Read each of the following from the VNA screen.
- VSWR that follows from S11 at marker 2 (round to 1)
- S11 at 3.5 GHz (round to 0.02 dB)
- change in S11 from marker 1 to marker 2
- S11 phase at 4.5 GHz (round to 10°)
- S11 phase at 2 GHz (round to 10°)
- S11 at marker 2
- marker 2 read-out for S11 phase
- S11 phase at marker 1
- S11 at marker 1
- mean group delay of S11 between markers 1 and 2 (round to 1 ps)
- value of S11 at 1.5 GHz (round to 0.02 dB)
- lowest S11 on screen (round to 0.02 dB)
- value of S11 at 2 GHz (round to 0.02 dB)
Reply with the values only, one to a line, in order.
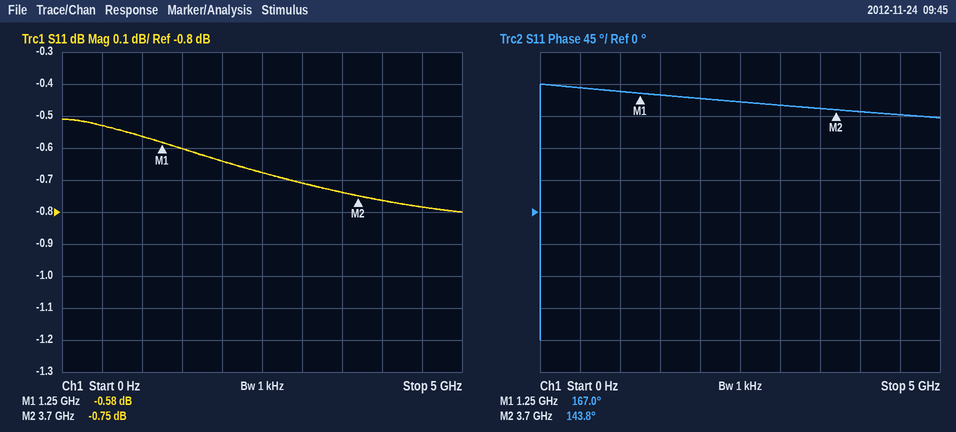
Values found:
23
-0.74 dB
-0.17 dB
140°
160°
-0.75 dB
143.8°
167.0°
-0.58 dB
26 ps
-0.60 dB
-0.80 dB
-0.64 dB
